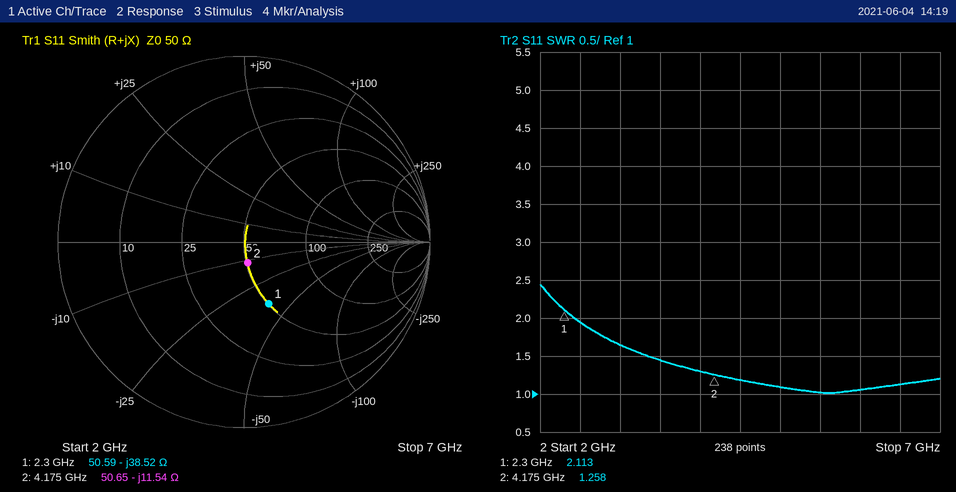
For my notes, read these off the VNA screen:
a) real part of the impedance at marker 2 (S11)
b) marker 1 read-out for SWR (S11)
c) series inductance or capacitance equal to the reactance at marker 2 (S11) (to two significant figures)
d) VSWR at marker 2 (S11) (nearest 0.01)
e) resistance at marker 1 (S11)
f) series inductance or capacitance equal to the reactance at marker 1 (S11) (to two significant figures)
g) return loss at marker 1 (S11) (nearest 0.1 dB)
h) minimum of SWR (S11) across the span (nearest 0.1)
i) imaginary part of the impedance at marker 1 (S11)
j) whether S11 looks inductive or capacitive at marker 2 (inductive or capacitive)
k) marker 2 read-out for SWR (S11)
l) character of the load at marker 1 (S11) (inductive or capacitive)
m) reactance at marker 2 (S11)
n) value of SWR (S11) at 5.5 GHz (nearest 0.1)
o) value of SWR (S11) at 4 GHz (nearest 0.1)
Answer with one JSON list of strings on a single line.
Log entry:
["50.65 Ω", "2.113", "3.3 pF", "1.26", "50.59 Ω", "1.8 pF", "8.9 dB", "1.0", "-38.52 Ω", "capacitive", "1.258", "capacitive", "-11.54 Ω", "1.0", "1.3"]
